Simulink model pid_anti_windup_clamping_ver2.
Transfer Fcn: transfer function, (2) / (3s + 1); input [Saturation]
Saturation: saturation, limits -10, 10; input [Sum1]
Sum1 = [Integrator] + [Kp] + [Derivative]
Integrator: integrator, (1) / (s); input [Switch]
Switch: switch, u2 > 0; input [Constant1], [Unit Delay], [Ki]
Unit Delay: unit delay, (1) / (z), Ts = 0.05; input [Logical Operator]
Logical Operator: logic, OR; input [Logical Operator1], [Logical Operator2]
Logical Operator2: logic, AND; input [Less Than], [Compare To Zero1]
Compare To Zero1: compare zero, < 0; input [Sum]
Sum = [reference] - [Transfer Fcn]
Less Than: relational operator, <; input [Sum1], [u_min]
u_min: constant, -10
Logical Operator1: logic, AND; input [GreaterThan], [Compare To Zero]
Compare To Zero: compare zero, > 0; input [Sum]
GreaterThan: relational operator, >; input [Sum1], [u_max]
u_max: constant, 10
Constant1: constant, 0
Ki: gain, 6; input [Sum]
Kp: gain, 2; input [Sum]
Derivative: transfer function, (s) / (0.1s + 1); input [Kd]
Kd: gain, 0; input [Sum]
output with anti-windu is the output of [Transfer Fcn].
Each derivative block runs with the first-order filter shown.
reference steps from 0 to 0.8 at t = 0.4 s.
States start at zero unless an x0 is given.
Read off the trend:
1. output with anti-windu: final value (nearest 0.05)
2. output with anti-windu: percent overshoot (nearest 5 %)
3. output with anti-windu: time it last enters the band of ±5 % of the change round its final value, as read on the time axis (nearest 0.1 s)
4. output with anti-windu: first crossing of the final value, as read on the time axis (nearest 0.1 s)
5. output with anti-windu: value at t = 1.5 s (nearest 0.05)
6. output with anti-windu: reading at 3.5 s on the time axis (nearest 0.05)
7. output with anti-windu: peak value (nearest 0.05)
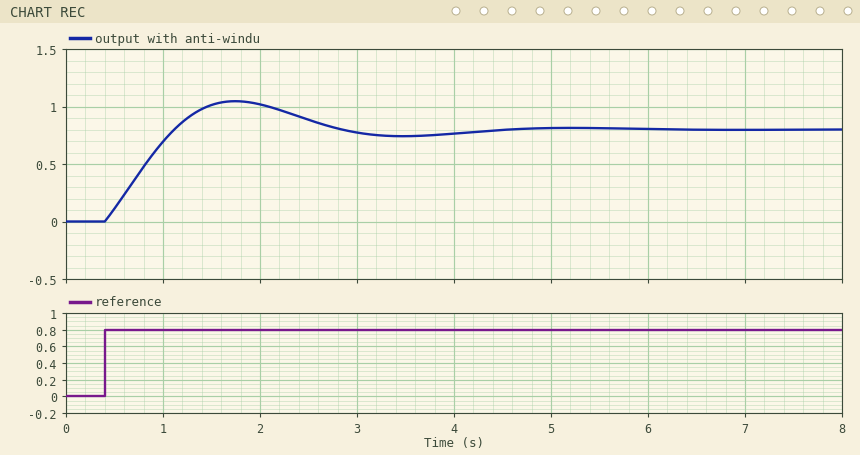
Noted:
0.80
30 %
3.9 s
1.1 s
1.00
0.75
1.05
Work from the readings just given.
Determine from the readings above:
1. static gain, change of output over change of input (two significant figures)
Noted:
1.0
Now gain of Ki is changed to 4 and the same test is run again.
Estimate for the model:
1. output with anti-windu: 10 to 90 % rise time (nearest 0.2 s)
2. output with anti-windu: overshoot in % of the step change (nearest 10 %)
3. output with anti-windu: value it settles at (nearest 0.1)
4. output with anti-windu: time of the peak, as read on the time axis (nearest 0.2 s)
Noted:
0.6 s
20 %
0.8
2.0 s
